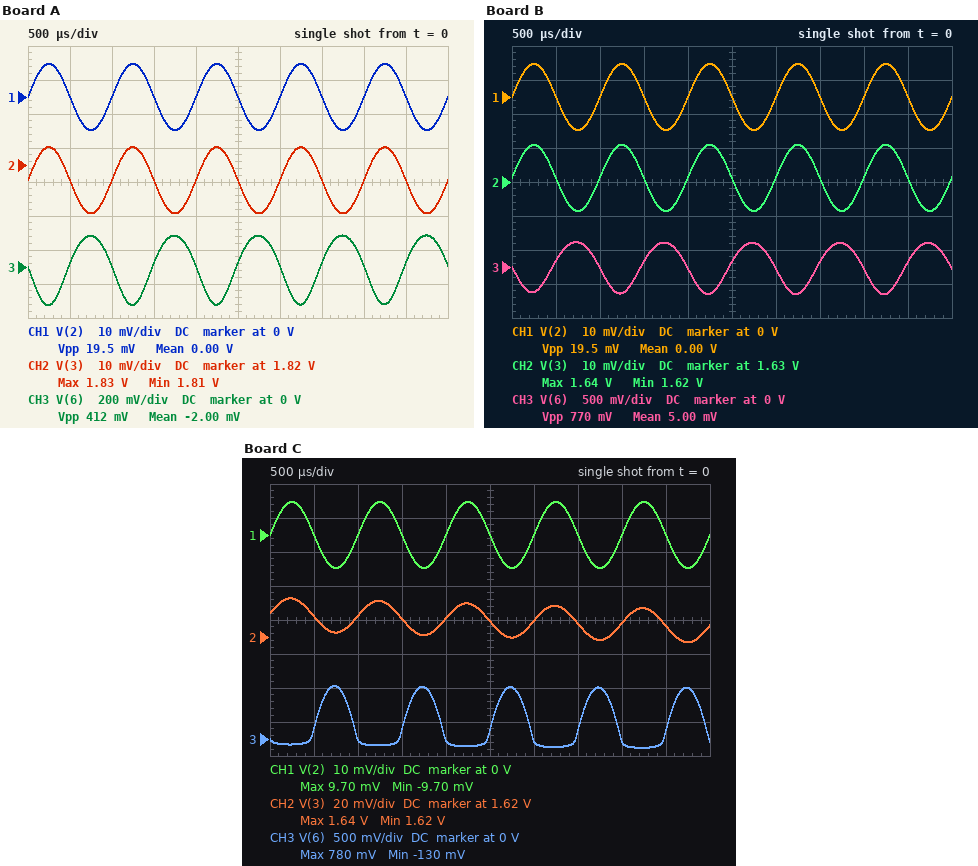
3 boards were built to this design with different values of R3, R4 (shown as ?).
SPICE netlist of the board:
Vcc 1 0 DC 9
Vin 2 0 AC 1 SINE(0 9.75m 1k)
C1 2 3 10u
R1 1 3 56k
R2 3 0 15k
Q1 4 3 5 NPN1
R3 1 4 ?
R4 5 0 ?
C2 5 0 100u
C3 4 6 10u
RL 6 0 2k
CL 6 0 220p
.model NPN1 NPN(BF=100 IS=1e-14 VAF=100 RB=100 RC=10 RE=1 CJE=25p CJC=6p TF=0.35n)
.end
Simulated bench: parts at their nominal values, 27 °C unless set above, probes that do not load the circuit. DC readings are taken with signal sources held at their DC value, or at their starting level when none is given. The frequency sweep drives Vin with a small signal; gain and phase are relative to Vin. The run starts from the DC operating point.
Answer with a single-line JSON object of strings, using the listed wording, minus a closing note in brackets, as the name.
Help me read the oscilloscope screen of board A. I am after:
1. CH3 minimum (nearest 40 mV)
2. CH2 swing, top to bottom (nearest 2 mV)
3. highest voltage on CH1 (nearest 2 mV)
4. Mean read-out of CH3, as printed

{"CH3 minimum": "-240 mV", "CH2 swing, top to bottom": "20 mV", "highest voltage on CH1": "10 mV", "Mean read-out of CH3, as printed": "-2.00 mV"}
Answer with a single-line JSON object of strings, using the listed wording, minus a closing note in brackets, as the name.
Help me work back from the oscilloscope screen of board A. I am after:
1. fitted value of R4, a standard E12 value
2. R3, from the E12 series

{"fitted value of R4, a standard E12 value": "1.5 kΩ", "R3, from the E12 series": "1.2 kΩ"}
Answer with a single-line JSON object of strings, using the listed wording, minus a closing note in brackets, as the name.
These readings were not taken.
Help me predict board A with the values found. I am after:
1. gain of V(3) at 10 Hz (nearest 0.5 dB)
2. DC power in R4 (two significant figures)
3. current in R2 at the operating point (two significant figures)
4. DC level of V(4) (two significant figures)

{"gain of V(3) at 10 Hz": "-1.0 dB", "DC power in R4": "910 µW", "current in R2 at the operating point": "120 µA", "DC level of V(4)": "8.1 V"}
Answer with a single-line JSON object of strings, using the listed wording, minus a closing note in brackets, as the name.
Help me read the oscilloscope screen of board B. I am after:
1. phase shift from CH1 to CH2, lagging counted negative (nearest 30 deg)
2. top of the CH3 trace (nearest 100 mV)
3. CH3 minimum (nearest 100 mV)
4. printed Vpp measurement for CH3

{"phase shift from CH1 to CH2, lagging counted negative": "0 deg", "top of the CH3 trace": "400 mV", "CH3 minimum": "-400 mV", "printed Vpp measurement for CH3": "770 mV"}
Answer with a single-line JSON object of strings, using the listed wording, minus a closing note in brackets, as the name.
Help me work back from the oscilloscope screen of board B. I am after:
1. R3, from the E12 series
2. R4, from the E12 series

{"R3, from the E12 series": "680 Ω", "R4, from the E12 series": "390 Ω"}
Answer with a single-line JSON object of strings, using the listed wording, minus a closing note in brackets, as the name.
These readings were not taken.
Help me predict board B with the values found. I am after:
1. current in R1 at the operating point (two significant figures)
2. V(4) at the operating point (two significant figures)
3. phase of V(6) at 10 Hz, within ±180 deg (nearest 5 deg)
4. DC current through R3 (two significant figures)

{"current in R1 at the operating point": "130 µA", "V(4) at the operating point": "7.4 V", "phase of V(6) at 10 Hz, within ±180 deg": "-75 deg", "DC current through R3": "2.4 mA"}
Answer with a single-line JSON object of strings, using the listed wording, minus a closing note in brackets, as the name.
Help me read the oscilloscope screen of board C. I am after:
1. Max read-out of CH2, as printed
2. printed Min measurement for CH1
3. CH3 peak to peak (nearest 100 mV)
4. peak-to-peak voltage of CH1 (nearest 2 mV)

{"Max read-out of CH2, as printed": "1.64 V", "printed Min measurement for CH1": "-9.70 mV", "CH3 peak to peak": "900 mV", "peak-to-peak voltage of CH1": "20 mV"}
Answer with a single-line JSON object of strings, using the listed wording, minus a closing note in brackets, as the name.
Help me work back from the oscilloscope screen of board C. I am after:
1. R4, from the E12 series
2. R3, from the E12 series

{"R4, from the E12 series": "470 Ω", "R3, from the E12 series": "3.9 kΩ"}
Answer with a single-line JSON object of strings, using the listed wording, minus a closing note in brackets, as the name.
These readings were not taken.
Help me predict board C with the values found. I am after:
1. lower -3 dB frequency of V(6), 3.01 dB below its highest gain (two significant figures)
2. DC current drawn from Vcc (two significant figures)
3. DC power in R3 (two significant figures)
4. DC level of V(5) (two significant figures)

{"lower -3 dB frequency of V(6), 3.01 dB below its highest gain": "130 Hz", "DC current drawn from Vcc": "2.1 mA", "DC power in R3": "16 mW", "DC level of V(5)": "960 mV"}
